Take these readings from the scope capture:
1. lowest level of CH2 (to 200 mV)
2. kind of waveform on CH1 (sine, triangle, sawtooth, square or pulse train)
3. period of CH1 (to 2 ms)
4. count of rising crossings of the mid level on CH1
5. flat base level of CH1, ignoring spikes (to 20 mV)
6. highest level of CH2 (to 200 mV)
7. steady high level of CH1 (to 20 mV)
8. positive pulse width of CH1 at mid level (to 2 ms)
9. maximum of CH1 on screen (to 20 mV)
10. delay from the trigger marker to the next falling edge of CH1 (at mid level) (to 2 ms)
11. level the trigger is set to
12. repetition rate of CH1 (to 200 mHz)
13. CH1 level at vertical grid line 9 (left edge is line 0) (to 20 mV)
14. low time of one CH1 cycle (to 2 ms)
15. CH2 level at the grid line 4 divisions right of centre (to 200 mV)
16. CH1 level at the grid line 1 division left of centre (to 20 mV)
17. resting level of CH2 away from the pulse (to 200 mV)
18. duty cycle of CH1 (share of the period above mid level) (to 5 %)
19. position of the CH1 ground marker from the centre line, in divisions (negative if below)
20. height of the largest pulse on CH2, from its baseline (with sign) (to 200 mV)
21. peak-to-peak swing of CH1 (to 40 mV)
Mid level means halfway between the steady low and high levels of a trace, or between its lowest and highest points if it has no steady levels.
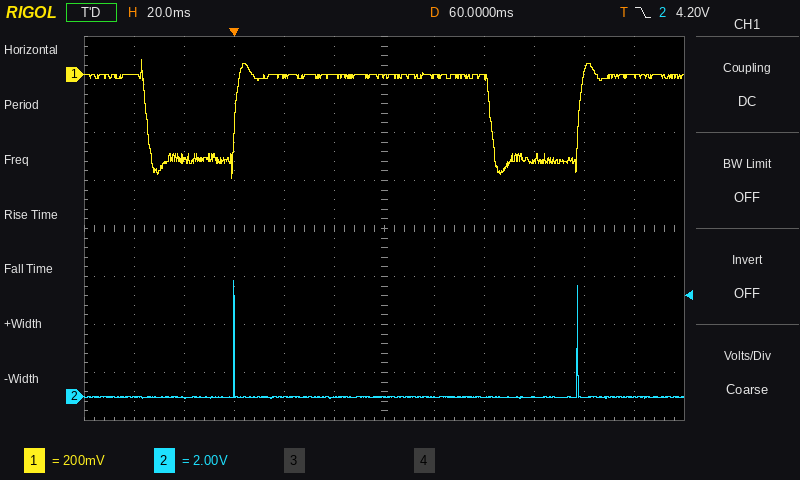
0.0 V
pulse train
138 ms
2
-360 mV
4.8 V
0 mV
102 ms
60 mV
102 ms
4.20 V
7.2 Hz
-340 mV
36 ms
0.0 V
0 mV
0.0 V
75 %
+3.2 div
+4.8 V
480 mV
